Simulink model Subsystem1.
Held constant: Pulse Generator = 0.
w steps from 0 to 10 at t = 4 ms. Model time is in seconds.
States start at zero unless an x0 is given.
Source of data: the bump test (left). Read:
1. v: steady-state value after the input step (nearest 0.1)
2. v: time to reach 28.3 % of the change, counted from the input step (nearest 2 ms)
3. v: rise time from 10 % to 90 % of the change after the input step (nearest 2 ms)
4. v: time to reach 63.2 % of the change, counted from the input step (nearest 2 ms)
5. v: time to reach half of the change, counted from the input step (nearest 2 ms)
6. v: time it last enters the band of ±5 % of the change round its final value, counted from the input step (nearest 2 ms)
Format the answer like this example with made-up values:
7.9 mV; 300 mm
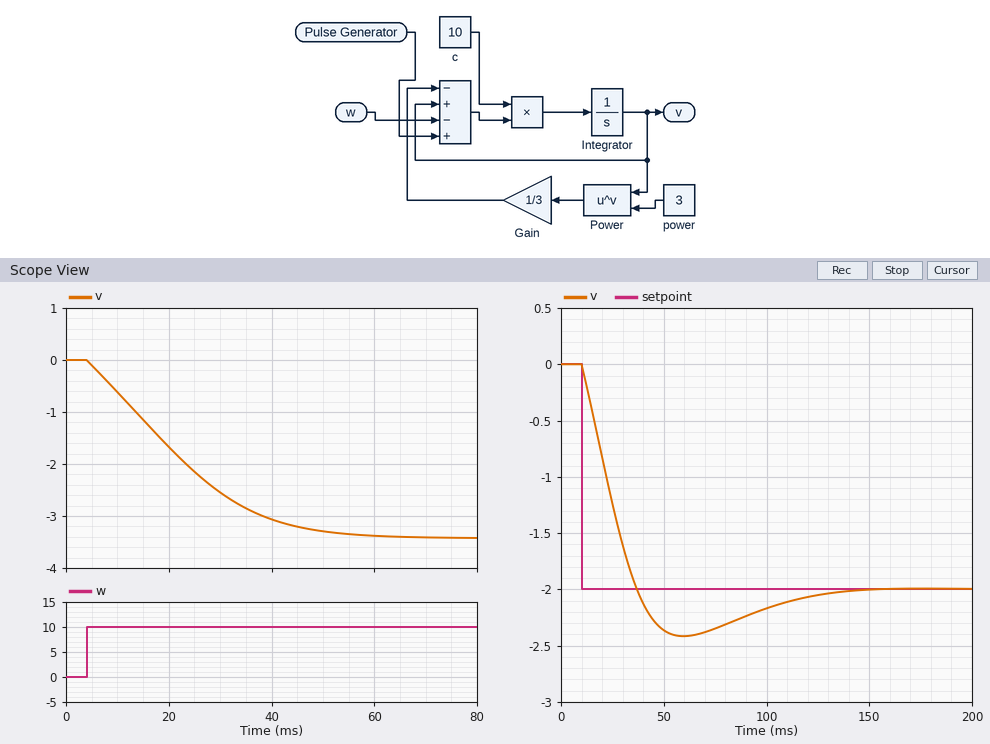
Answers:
-3.4; 10 ms; 34 ms; 22 ms; 16 ms; 44 ms
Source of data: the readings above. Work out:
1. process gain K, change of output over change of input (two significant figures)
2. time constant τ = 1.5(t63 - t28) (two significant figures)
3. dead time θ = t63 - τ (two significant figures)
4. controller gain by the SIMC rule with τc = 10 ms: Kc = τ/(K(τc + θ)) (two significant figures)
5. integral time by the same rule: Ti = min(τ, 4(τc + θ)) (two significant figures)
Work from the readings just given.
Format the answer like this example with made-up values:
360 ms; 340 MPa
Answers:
-0.34; 18 ms; 4.0 ms; -3.8; 18 ms
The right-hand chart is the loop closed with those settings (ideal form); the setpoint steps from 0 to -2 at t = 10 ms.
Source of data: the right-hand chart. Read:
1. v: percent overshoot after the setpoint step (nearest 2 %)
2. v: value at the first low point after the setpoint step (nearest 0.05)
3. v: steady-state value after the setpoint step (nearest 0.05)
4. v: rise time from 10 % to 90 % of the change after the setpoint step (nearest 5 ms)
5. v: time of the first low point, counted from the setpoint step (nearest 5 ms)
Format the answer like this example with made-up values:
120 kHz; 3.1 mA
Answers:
20 %; -2.40; -2.00; 20 ms; 50 ms
